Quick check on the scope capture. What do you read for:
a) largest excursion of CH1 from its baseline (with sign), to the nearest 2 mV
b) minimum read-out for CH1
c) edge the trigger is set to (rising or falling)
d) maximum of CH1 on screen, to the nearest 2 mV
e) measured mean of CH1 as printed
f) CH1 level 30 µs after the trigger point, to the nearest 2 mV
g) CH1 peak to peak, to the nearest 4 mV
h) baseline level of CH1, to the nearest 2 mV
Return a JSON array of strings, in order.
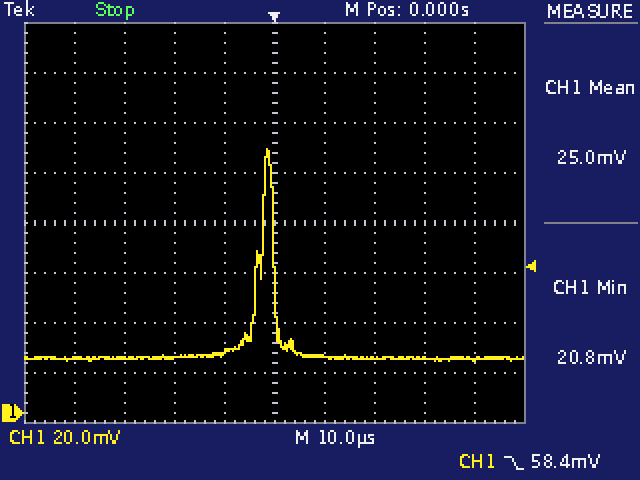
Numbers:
["+84 mV", "20.8 mV", "falling", "106 mV", "25.0 mV", "22 mV", "84 mV", "22 mV"]
